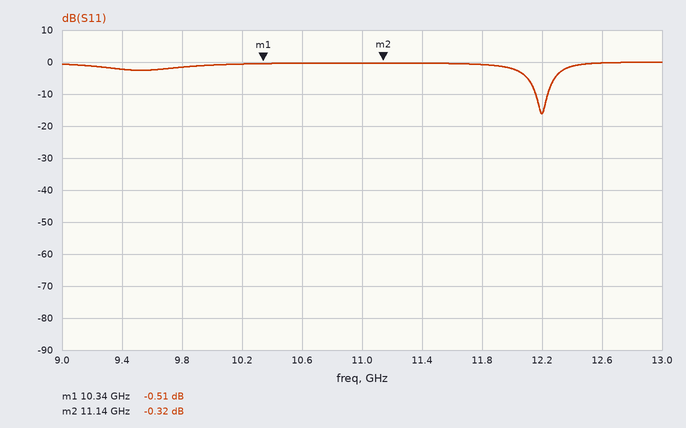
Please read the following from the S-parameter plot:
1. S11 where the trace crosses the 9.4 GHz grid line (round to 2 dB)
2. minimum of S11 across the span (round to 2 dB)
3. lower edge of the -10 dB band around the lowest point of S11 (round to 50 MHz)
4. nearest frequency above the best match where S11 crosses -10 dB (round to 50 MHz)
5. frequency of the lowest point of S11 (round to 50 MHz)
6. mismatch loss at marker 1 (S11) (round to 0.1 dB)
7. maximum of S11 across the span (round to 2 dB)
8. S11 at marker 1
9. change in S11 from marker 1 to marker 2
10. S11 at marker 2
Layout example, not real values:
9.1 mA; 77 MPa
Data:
-2 dB; -16 dB; 12.15 GHz; 12.25 GHz; 12.20 GHz; 9.6 dB; 0 dB; -0.51 dB; 0.19 dB; -0.32 dB
